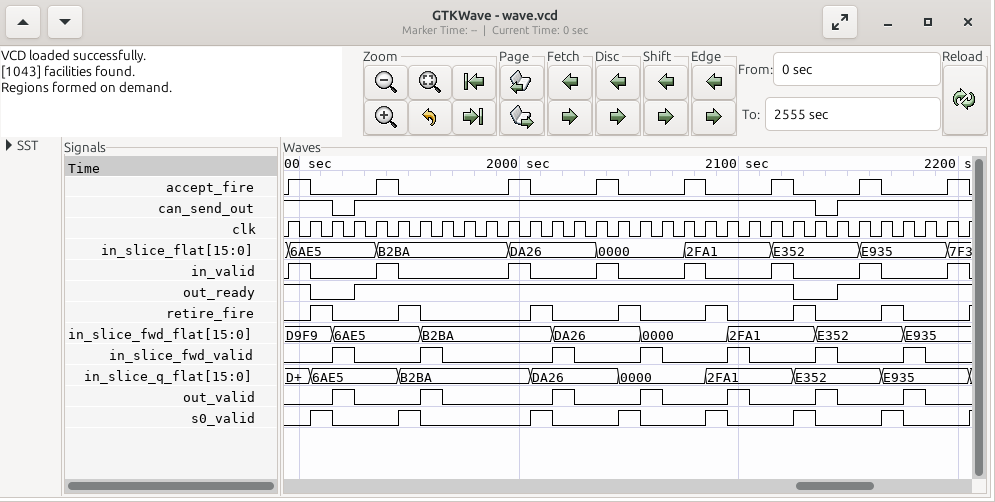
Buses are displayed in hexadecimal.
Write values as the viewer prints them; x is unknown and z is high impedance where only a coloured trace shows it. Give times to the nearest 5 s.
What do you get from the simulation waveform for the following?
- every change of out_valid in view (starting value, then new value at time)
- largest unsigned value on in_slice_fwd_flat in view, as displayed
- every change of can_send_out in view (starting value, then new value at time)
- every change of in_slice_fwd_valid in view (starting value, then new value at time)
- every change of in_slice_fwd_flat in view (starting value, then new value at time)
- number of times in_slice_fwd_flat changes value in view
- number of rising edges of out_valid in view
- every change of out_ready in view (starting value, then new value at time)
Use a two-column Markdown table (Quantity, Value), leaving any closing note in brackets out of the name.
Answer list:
| Quantity | Value |
|---|---|
| every change of out_valid in view | 0, 1 at 1915 s, 0 at 1925 s, 1 at 1955 s, 0 at 1965 s, 1 at 2015 s, 0 at 2025 s, 1 at 2055 s, 0 at 2065 s, 1 at 2095 s, 0 at 2105 s, 1 at 2135 s, 0 at 2145 s, 1 at 2175 s, 0 at 2185 s |
| largest unsigned value on in_slice_fwd_flat in view, as displayed | E935 |
| every change of can_send_out in view | 1, 0 at 1915 s, 1 at 1925 s, 0 at 2135 s, 1 at 2145 s |
| every change of in_slice_fwd_valid in view | 0, 1 at 1915 s, 0 at 1925 s, 1 at 1955 s, 0 at 1965 s, 1 at 2015 s, 0 at 2025 s, 1 at 2055 s, 0 at 2065 s, 1 at 2095 s, 0 at 2105 s, 1 at 2135 s, 0 at 2145 s, 1 at 2175 s, 0 at 2185 s |
| every change of in_slice_fwd_flat in view | D9F9, 6AE5 at 1915 s, B2BA at 1955 s, DA26 at 2015 s, 0000 at 2055 s, 2FA1 at 2095 s, E352 at 2135 s, E935 at 2175 s |
| number of times in_slice_fwd_flat changes value in view | 7 |
| number of rising edges of out_valid in view | 7 |
| every change of out_ready in view | 1, 0 at 1905 s, 1 at 1925 s, 0 at 2125 s, 1 at 2145 s |
